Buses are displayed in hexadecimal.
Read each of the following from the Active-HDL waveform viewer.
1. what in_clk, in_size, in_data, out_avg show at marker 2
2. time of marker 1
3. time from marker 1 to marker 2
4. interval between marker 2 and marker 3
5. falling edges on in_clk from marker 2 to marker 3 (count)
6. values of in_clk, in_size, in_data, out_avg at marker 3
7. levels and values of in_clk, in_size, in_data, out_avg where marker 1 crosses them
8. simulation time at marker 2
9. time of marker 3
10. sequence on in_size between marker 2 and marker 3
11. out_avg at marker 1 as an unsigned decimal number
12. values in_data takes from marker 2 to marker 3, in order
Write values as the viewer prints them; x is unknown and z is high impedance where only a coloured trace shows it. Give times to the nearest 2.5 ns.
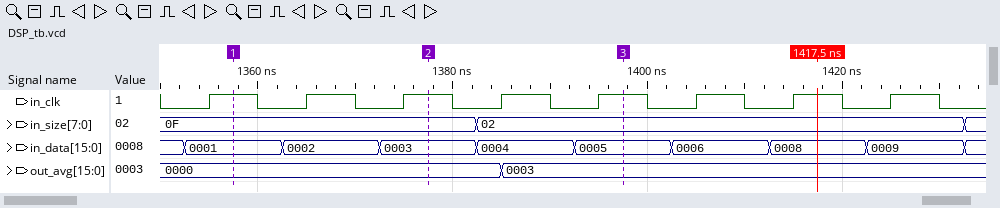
in_clk=1, in_size=0F, in_data=0003, out_avg=0000
1357.5 ns
20 ns
20 ns
2
in_clk=1, in_size=02, in_data=0005, out_avg=0003
in_clk=1, in_size=0F, in_data=0001, out_avg=0000
1377.5 ns
1397.5 ns
0F, 02
0
0003, 0004, 0005
